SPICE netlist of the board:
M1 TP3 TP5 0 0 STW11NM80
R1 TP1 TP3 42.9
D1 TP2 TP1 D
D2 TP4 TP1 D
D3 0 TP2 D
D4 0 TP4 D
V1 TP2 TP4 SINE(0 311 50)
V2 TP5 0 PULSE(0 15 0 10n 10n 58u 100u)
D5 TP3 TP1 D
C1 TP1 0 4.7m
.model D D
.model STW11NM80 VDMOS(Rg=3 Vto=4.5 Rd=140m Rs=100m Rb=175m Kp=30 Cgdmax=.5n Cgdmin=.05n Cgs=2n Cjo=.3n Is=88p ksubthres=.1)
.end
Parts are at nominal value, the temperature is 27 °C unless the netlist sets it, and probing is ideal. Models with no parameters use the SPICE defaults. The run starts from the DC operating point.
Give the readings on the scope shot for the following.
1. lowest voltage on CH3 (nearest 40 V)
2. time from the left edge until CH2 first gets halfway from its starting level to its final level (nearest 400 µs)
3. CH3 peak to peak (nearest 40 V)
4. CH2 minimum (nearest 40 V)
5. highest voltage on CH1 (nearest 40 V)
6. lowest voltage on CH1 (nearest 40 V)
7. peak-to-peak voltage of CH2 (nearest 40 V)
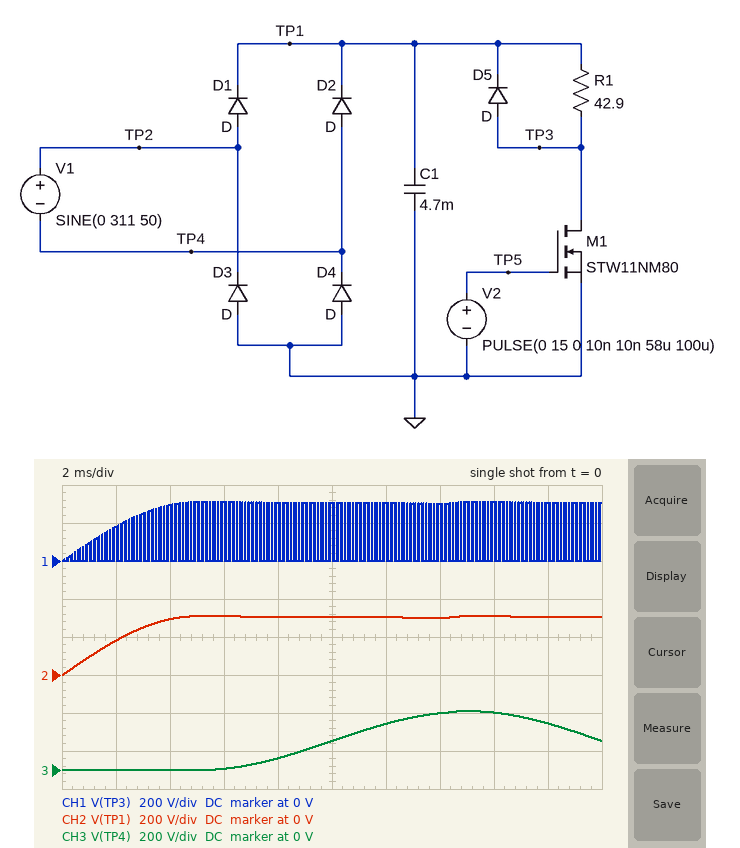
0 V
1.6 ms
320 V
0 V
320 V
0 V
320 V
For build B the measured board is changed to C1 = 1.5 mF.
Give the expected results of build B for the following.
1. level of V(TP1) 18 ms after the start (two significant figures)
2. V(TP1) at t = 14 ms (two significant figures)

300 V
290 V
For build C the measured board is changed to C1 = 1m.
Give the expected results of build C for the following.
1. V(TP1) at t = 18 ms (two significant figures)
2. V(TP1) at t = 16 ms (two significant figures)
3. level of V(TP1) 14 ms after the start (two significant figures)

300 V
310 V
290 V
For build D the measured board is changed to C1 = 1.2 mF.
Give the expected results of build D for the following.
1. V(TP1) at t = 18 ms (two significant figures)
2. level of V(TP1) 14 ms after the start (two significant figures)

300 V
290 V
